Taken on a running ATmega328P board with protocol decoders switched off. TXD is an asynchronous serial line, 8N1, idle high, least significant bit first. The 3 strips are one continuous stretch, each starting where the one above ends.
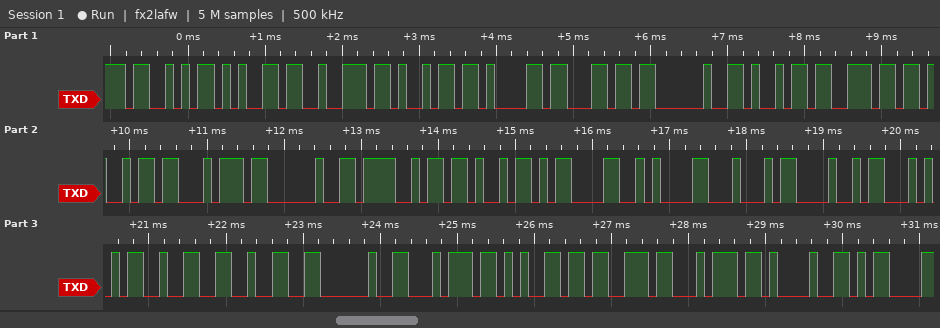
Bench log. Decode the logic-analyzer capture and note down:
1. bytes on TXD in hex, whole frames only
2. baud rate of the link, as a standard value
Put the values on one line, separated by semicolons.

53 65 72 69 61 6C 20 69 6E 69 74 20 4F 4B 0D 0A 44 48 54 32 32 20 74 65 73 74 21 0D; 9600 baud
